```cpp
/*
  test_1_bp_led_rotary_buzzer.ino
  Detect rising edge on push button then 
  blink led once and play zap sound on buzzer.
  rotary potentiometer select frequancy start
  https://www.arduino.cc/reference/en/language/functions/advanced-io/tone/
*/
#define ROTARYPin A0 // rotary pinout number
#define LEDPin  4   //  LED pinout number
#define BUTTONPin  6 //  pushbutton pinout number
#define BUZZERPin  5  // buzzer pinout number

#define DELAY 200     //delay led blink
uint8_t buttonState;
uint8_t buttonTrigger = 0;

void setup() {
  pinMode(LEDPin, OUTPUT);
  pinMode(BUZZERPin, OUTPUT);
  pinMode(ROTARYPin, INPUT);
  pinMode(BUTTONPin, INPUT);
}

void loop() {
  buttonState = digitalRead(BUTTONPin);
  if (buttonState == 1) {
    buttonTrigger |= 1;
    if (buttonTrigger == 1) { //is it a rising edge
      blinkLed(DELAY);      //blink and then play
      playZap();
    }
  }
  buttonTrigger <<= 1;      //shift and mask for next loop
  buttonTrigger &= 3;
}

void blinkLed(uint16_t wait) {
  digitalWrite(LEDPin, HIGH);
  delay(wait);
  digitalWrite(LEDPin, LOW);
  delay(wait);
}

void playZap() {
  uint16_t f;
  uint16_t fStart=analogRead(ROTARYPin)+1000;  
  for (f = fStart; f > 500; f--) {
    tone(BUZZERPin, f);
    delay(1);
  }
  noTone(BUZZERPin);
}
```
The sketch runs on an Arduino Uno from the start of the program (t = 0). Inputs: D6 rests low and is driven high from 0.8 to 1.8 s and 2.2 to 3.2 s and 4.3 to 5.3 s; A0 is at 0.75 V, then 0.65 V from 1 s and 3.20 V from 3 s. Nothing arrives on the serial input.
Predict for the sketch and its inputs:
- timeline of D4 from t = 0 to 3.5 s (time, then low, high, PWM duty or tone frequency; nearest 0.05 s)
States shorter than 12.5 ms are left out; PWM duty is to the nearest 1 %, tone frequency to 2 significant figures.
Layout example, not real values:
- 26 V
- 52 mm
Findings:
- 0 s low; 0.8 s high; 1 s low; 2.2 s high; 2.4 s low
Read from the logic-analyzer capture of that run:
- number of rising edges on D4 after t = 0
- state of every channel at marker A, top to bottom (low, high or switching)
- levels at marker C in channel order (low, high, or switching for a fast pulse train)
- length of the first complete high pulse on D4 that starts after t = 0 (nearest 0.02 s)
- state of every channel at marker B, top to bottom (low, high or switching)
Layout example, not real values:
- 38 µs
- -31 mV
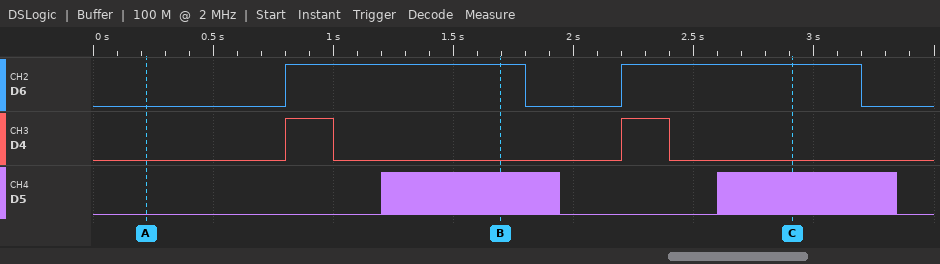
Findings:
- 2
- D6 low, D4 low, D5 low
- D6 high, D4 low, D5 switching
- 0.20 s
- D6 high, D4 low, D5 switching
